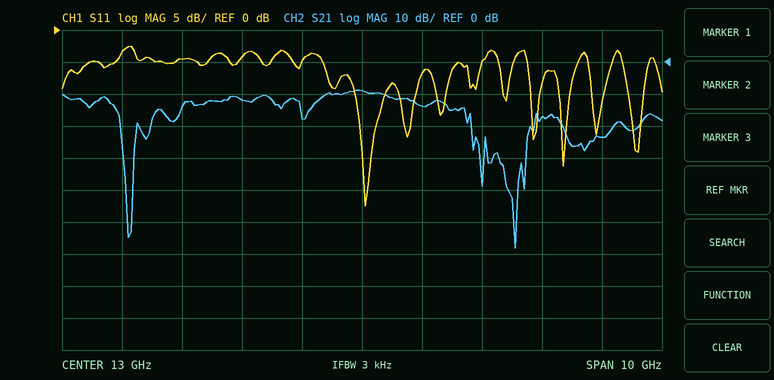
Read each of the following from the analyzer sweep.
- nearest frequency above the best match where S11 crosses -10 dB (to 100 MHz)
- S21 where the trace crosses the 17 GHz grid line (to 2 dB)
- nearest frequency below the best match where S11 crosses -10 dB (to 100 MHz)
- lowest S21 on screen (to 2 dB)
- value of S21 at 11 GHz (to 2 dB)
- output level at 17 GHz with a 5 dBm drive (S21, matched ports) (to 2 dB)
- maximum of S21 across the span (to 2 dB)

13.4 GHz
-24 dB
12.9 GHz
-58 dB
-12 dB
-18 dBm
-8 dB
